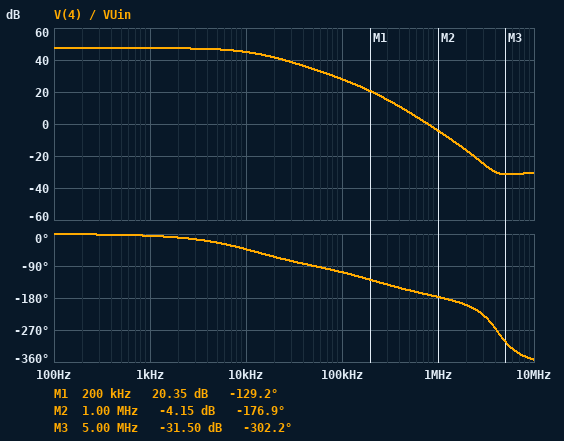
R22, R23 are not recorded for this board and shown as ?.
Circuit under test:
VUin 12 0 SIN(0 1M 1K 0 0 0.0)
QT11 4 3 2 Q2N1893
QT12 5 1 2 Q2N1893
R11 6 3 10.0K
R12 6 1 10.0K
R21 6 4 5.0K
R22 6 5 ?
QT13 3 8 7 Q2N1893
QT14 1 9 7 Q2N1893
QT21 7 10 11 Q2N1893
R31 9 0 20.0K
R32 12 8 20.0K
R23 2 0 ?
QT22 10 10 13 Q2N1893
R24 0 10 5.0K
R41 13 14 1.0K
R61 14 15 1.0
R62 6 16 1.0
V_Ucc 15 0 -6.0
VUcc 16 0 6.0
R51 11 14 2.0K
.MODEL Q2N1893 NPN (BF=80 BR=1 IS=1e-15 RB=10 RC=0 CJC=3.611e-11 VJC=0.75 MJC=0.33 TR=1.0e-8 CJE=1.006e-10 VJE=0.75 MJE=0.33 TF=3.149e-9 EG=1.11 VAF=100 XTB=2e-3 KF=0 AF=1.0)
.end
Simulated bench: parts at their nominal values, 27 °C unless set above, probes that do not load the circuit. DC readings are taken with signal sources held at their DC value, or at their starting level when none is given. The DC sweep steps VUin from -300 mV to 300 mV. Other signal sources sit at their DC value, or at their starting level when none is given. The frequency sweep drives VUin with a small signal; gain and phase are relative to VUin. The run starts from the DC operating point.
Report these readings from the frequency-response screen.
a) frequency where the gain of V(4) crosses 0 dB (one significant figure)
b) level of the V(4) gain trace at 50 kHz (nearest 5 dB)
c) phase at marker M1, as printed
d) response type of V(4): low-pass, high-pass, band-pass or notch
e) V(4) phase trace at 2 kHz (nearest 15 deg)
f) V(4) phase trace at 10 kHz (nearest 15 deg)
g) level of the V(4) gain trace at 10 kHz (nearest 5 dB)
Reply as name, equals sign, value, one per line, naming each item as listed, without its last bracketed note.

frequency where the gain of V(4) crosses 0 dB = 800 kHz
level of the V(4) gain trace at 50 kHz = 35 dB
phase at marker M1, as printed = -129.2 deg
response type of V(4): low-pass, high-pass, band-pass or notch = low-pass
V(4) phase trace at 2 kHz = -15 deg
V(4) phase trace at 10 kHz = -45 deg
level of the V(4) gain trace at 10 kHz = 45 dB
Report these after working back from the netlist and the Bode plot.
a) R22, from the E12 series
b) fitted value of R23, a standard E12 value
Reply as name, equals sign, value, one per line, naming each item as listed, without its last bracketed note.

R22, from the E12 series = 6.8 kΩ
fitted value of R23, a standard E12 value = 10 kΩ
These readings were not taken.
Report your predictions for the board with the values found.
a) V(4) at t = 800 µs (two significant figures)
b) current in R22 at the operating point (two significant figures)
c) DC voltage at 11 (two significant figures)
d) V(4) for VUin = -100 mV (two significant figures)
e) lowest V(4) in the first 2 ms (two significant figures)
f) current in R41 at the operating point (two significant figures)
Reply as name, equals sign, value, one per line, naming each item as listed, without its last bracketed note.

V(4) at t = 800 µs = 5.0 V
current in R22 at the operating point = 150 µA
DC voltage at 11 = -5.1 V
V(4) for VUin = -100 mV = 4.1 V
lowest V(4) in the first 2 ms = 5.0 V
current in R41 at the operating point = 880 µA
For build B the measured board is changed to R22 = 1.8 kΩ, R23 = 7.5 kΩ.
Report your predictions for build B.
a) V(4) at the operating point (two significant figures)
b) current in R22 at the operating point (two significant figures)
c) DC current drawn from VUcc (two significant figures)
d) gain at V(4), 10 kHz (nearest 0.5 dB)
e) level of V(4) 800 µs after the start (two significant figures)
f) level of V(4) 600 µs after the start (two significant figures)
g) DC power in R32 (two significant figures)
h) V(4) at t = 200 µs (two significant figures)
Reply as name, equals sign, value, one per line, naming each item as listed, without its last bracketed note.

V(4) at the operating point = 5.0 V
current in R22 at the operating point = 210 µA
DC current drawn from VUcc = 850 µA
gain at V(4), 10 kHz = 47.0 dB
level of V(4) 800 µs after the start = 4.7 V
level of V(4) 600 µs after the start = 4.8 V
DC power in R32 = 140 nW
V(4) at t = 200 µs = 5.2 V
